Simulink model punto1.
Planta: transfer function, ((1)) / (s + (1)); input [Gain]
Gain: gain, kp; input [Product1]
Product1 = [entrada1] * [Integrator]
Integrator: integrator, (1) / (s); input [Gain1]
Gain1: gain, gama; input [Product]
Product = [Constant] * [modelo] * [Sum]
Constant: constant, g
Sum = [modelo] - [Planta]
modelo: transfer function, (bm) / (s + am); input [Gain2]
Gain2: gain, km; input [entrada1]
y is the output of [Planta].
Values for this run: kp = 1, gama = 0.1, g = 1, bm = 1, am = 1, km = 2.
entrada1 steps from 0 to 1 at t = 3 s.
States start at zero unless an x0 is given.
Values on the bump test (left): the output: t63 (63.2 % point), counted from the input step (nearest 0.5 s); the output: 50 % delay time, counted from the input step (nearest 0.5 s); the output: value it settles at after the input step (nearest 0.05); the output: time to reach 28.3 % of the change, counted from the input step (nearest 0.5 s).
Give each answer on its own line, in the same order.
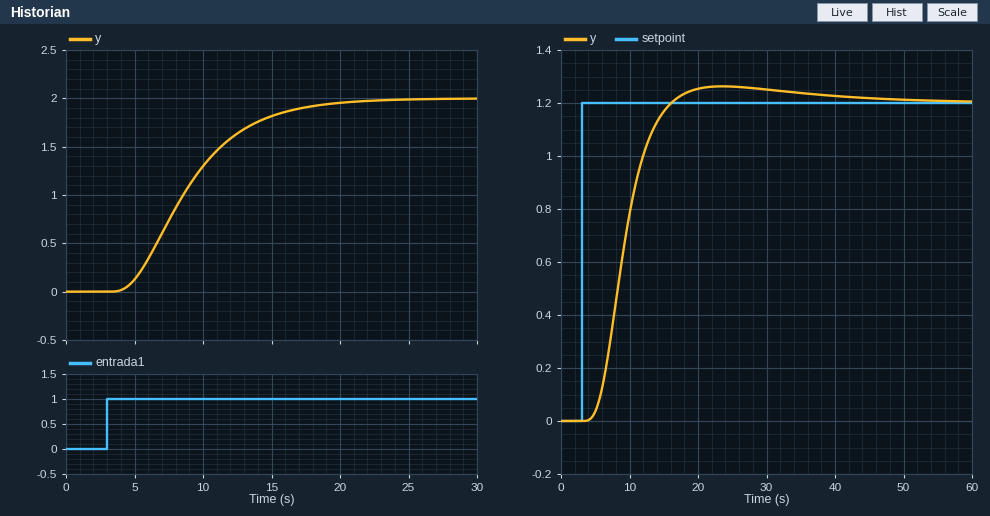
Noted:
7.0 s
5.5 s
2.00
4.0 s
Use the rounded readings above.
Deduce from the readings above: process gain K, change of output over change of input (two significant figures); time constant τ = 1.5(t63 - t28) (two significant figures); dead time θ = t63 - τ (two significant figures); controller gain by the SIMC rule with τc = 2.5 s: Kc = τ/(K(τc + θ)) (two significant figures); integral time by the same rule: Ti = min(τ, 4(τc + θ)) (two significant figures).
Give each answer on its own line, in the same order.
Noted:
2.0
4.5 s
2.5 s
0.45
4.5 s
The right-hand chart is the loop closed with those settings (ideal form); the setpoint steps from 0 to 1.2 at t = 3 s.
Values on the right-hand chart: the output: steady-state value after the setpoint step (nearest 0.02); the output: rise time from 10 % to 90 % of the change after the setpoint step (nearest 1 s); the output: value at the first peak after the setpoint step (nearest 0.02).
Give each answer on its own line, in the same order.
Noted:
1.20
7 s
1.26
